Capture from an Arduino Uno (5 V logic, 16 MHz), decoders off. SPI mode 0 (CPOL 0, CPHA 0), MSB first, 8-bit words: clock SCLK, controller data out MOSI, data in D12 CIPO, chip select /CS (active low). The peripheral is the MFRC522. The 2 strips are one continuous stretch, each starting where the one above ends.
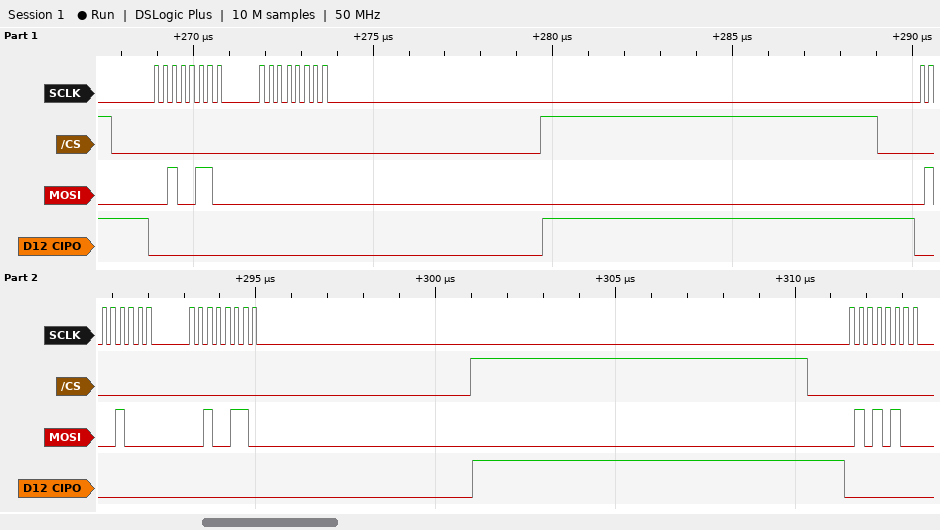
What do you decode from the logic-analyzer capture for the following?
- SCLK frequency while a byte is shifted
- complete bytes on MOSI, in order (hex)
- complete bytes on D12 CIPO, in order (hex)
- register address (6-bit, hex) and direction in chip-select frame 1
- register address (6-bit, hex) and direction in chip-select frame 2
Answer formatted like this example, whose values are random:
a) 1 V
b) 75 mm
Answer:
a) 4 MHz
b) 26 00 48 26 54
c) 00 00 00 00 00
d) 0x13 write
e) 0x24 write
